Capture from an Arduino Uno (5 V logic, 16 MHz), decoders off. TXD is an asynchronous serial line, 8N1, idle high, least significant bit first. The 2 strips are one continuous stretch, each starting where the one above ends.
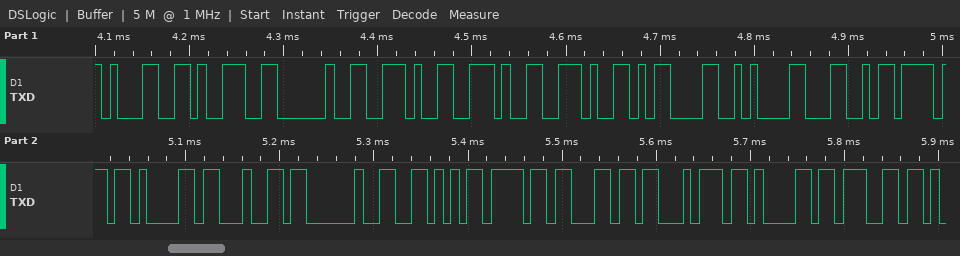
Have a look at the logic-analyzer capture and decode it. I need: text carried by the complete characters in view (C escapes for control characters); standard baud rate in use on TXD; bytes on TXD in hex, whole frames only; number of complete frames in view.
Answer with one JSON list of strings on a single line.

["\"19 ...\\r\\nLoad Voltag\"", "115200 baud", "31 39 20 2E 2E 2E 0D 0A 4C 6F 61 64 20 56 6F 6C 74 61 67", "19"]
